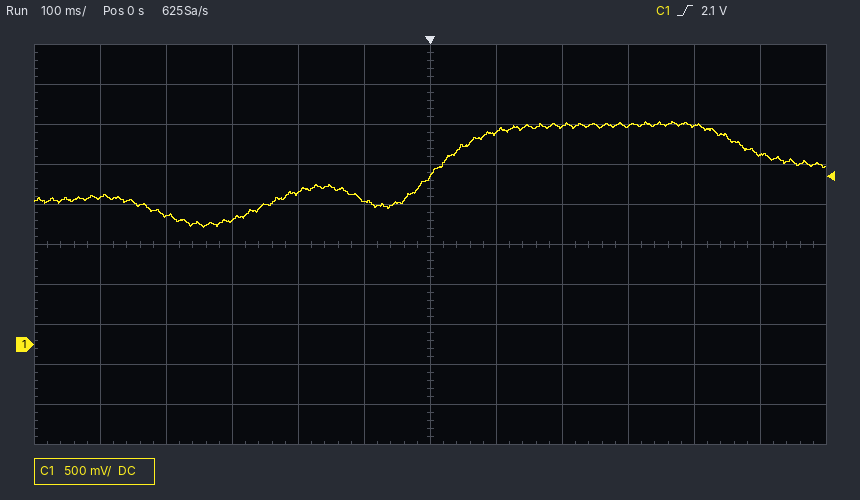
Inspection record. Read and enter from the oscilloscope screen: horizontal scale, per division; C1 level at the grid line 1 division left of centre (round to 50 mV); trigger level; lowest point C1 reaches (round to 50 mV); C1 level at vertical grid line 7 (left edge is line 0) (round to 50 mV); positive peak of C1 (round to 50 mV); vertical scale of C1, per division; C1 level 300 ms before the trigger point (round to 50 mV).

100 ms
1.80 V
2.1 V
1.45 V
2.65 V
2.80 V
500 mV
1.55 V
